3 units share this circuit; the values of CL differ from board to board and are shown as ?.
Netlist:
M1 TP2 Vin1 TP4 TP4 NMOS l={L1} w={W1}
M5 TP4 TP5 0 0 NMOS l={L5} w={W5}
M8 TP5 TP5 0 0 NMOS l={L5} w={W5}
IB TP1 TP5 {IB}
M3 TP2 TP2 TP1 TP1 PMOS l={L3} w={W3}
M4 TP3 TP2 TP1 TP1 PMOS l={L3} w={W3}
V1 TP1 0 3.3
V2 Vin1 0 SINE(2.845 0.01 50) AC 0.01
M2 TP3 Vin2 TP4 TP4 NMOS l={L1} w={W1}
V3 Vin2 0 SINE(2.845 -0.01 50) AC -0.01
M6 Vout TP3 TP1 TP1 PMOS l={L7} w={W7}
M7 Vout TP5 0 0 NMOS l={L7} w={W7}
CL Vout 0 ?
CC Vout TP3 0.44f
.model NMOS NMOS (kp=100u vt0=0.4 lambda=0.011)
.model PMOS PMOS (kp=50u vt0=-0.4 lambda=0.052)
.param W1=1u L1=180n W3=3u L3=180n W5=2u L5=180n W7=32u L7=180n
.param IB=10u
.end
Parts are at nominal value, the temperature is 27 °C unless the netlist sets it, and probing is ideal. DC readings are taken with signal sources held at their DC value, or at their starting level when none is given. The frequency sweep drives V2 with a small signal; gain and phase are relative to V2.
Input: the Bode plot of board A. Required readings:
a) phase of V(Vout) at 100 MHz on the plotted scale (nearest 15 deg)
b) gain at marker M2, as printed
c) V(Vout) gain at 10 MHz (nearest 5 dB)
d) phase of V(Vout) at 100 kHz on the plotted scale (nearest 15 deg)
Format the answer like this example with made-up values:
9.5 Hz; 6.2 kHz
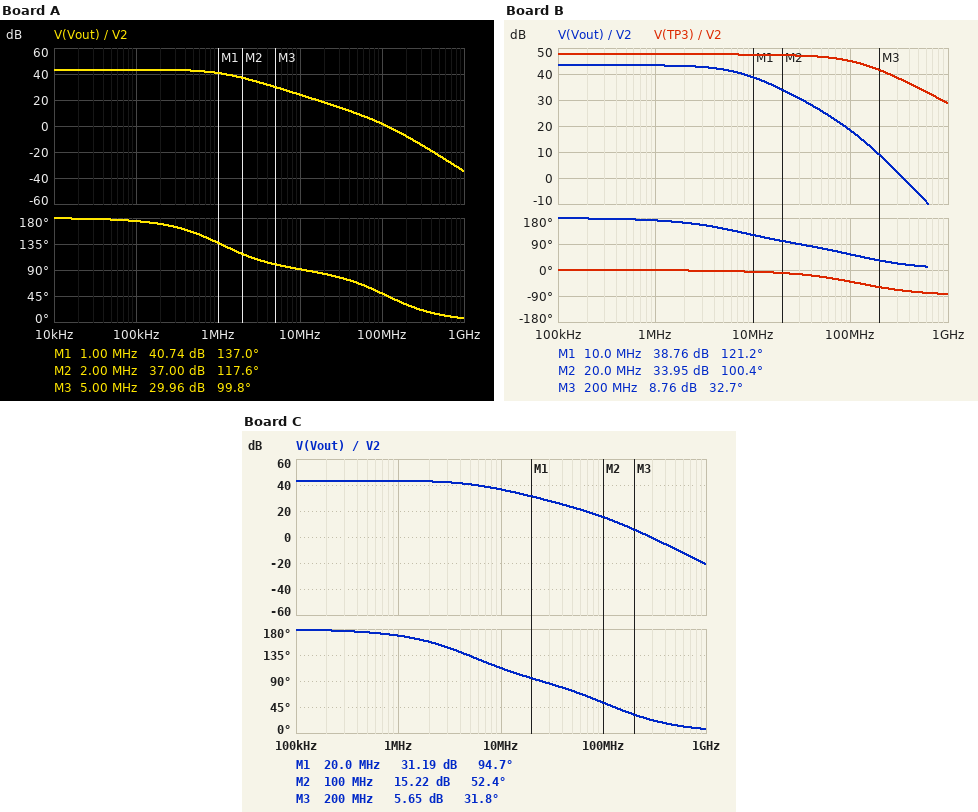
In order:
45 deg; 37.00 dB; 25 dB; 180 deg
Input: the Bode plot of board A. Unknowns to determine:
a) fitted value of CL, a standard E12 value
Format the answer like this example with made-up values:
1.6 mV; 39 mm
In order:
270 pF
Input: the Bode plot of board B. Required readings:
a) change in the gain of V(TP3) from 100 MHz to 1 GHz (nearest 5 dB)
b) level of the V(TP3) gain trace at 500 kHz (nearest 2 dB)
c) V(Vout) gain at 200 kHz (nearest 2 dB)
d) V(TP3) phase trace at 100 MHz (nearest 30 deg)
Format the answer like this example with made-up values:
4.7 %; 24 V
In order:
-15 dB; 48 dB; 44 dB; -30 deg
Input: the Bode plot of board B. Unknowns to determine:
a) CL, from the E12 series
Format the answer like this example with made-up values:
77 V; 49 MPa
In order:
39 pF
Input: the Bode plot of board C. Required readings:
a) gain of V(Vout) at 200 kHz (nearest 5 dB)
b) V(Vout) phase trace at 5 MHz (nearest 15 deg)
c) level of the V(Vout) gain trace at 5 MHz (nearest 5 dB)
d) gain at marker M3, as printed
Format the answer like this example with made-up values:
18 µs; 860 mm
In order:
45 dB; 135 deg; 40 dB; 5.65 dB
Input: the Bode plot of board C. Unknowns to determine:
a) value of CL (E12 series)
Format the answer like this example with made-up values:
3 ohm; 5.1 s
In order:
56 pF
